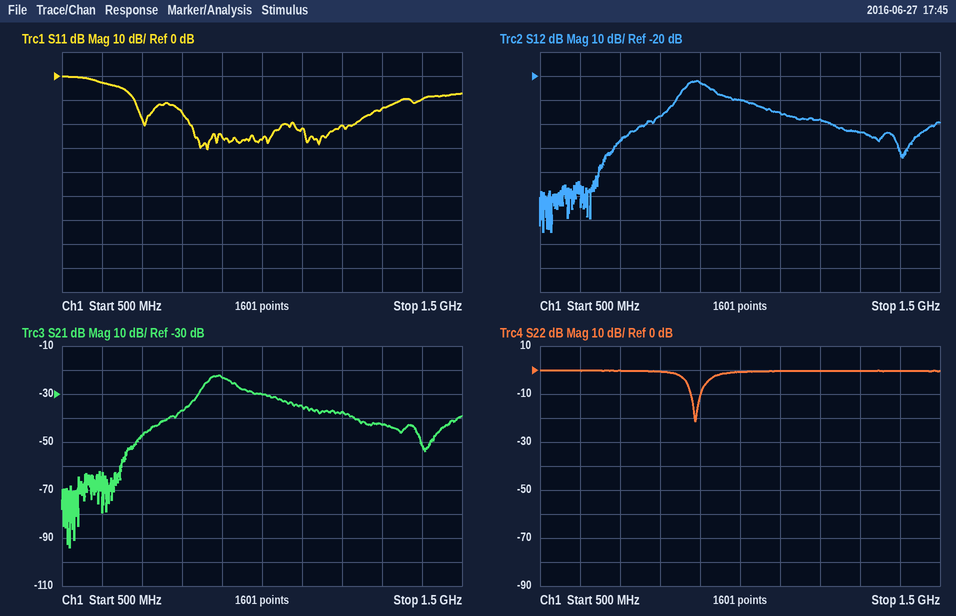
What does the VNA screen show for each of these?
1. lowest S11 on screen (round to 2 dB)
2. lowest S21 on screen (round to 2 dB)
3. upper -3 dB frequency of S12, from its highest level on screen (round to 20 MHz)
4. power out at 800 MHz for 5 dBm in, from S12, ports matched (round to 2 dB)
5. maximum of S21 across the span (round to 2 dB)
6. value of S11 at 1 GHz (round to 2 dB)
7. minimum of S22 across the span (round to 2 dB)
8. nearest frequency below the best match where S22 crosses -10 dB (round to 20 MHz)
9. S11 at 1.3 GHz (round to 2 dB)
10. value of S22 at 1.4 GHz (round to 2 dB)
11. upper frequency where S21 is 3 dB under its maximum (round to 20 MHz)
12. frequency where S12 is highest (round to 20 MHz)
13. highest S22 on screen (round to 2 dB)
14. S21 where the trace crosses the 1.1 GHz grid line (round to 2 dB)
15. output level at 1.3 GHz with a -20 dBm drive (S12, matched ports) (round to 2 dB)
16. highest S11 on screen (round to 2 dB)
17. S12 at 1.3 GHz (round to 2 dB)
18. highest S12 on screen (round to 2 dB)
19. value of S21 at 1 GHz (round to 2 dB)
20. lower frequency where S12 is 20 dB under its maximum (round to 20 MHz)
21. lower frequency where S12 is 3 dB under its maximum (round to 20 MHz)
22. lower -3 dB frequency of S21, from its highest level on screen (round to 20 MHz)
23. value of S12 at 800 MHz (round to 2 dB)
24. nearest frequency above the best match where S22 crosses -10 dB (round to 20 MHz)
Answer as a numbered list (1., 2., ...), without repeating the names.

1. -30 dB
2. -94 dB
3. 920 MHz
4. -32 dBm
5. -22 dB
6. -26 dB
7. -22 dB
8. 880 MHz
9. -14 dB
10. 0 dB
11. 920 MHz
12. 900 MHz
13. 0 dB
14. -36 dB
15. -64 dBm
16. 0 dB
17. -44 dB
18. -22 dB
19. -30 dB
20. 740 MHz
21. 860 MHz
22. 860 MHz
23. -36 dB
24. 900 MHz
